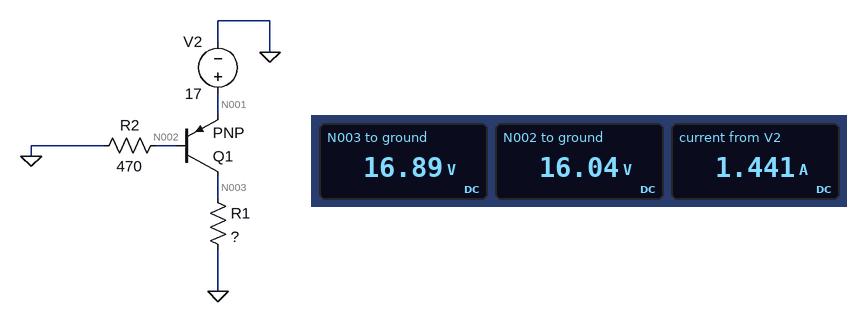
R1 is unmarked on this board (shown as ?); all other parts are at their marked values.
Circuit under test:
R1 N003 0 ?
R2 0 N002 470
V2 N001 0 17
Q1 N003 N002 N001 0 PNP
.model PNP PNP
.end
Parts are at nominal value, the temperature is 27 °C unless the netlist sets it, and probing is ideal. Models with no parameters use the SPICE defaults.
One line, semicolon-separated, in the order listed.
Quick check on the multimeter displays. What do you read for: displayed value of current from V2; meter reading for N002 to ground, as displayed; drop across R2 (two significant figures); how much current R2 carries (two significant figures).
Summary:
1.441 A; 16.04 V; 16 V; 34 mA
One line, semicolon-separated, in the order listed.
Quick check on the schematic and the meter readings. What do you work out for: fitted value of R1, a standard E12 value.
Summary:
12 Ω
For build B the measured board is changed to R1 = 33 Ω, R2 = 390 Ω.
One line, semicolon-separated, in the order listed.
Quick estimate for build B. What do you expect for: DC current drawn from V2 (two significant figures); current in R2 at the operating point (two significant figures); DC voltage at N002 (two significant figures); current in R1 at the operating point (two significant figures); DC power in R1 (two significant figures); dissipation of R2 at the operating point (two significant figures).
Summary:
550 mA; 41 mA; 16 V; 510 mA; 8.7 W; 660 mW
